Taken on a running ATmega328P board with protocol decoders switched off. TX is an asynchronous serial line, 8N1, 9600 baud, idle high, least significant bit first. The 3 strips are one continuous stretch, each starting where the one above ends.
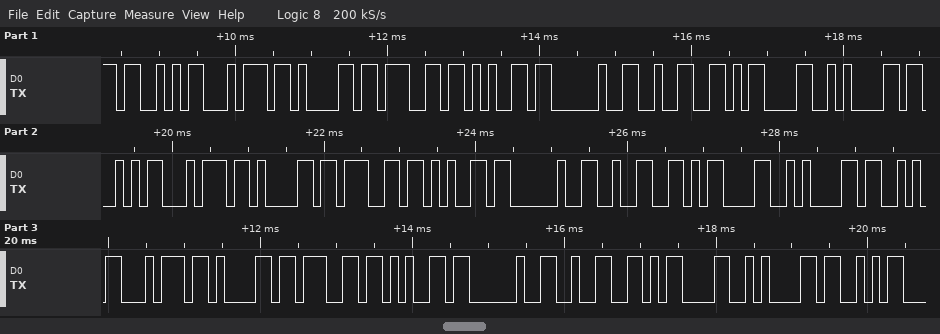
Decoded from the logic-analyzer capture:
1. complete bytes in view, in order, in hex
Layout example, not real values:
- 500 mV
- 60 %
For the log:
- 53 74 61 67 65 20 32 0D 0A 53 74 61 67 65 20 32 0D 0A 53 74 61 67 65 20 32 0D 0A 53
